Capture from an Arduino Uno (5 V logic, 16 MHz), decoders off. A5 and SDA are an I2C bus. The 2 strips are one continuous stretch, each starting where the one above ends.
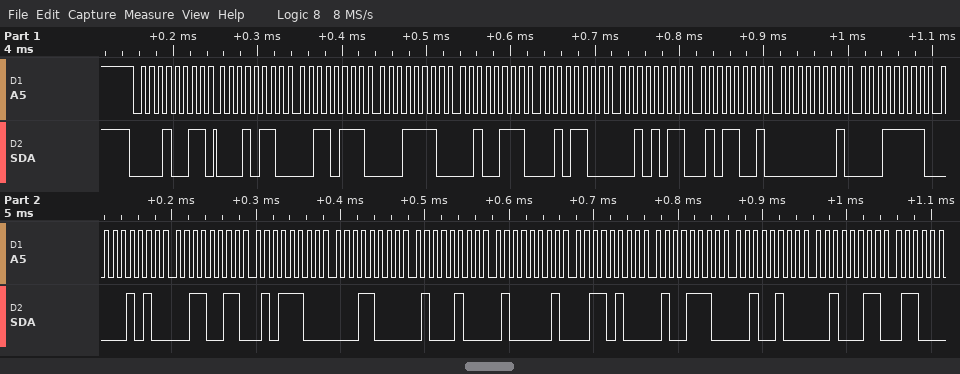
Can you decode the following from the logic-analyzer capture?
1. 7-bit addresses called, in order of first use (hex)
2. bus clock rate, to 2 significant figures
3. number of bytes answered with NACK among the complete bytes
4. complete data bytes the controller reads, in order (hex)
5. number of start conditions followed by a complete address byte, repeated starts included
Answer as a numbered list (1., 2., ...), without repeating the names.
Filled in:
1. 0x09
2. 100 kHz
3. 0
4. 16 37 1E 27 2C 2B 59 01 1F 0A 33 5C 18 44 41 34 4E 24 23
5. 1
